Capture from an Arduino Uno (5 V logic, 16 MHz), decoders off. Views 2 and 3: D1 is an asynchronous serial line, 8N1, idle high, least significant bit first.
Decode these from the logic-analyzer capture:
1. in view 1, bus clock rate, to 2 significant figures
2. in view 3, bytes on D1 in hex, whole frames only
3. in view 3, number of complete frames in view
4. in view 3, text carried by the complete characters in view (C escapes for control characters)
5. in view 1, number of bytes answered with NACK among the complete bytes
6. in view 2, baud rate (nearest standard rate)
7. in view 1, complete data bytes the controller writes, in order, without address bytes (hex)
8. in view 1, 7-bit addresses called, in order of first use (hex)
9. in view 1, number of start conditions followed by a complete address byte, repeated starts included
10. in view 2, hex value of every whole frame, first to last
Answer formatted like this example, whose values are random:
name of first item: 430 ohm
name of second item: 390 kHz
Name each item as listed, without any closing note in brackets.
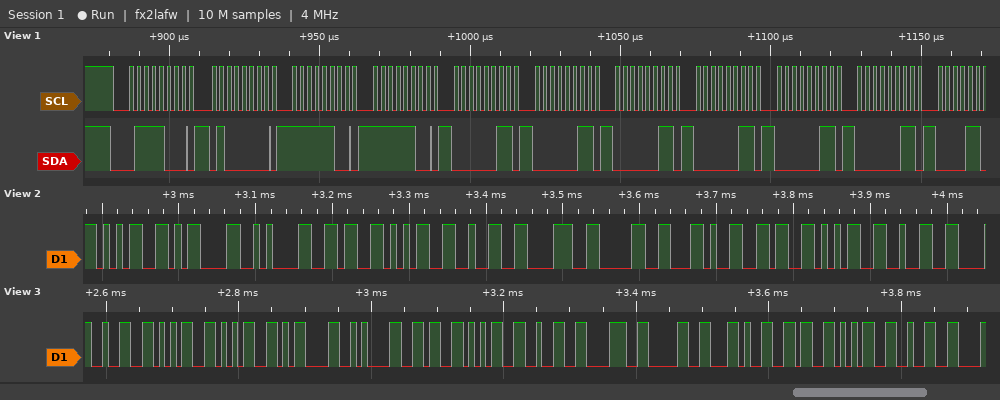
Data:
in view 1, bus clock rate, to 2 significant figures: 400 kHz
in view 3, bytes on D1 in hex, whole frames only: 0x32 0x35 0x35 0x0D 0x0A 0x36 0x35 0x32 0x38 0x30 0x2C 0x36 0x35 0x32
in view 3, number of complete frames in view: 14
in view 3, text carried by the complete characters in view: "255\r\n65280,652"
in view 1, number of bytes answered with NACK among the complete bytes: 0
in view 2, baud rate: 115200 baud
in view 1, complete data bytes the controller writes, in order, without address bytes: 40 FC FC 03 03 03 03 03 03
in view 1, 7-bit addresses called, in order of first use: 0x3C
in view 1, number of start conditions followed by a complete address byte, repeated starts included: 1
in view 2, hex value of every whole frame, first to last: 35 0D 0A 36 35 32 38 30 2C 36 35 32
